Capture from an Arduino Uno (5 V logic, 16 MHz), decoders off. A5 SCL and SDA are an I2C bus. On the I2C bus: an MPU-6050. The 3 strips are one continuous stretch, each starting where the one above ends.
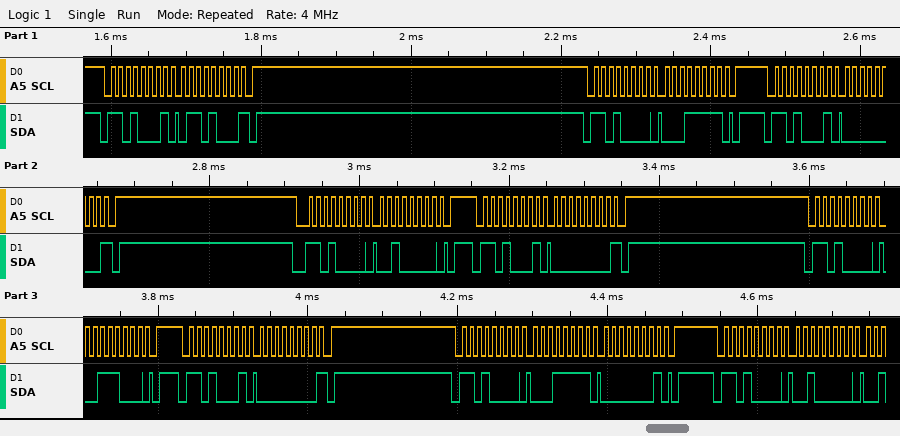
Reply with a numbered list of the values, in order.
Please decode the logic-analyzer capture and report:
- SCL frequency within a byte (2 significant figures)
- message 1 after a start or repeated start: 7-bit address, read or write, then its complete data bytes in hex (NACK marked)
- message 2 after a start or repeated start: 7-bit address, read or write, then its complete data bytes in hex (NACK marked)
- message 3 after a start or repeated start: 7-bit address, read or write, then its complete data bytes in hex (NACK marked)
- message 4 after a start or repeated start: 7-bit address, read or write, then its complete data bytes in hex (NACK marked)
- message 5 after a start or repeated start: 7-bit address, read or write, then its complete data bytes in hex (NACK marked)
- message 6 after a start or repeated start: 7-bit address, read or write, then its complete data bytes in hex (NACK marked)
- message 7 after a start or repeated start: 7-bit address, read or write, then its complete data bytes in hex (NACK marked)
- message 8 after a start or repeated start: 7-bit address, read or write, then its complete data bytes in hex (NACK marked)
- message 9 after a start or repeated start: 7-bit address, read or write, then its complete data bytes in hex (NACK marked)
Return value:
1. 100 kHz
2. 0x68 read: 68 NACK
3. 0x68 write: 1F
4. 0x68 read: 00 NACK
5. 0x68 write: 20
6. 0x68 read: 00 NACK
7. 0x68 write: 38
8. 0x68 read: 00 NACK
9. 0x68 write: 1F 01
10. 0x68 write: 20
